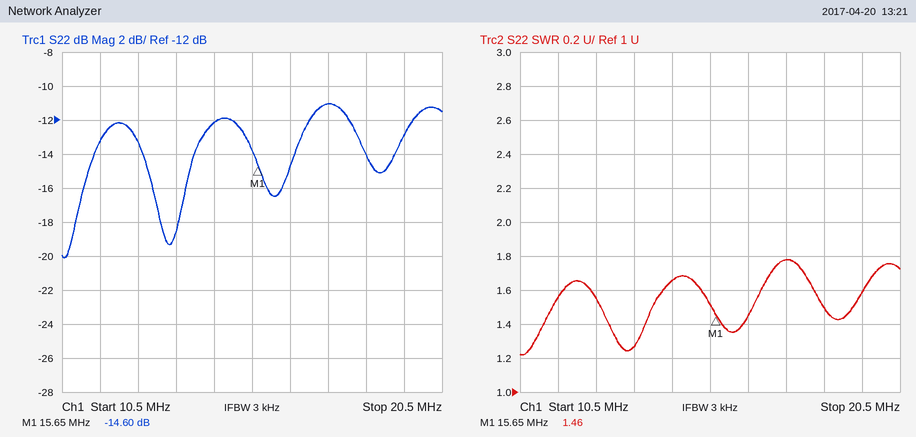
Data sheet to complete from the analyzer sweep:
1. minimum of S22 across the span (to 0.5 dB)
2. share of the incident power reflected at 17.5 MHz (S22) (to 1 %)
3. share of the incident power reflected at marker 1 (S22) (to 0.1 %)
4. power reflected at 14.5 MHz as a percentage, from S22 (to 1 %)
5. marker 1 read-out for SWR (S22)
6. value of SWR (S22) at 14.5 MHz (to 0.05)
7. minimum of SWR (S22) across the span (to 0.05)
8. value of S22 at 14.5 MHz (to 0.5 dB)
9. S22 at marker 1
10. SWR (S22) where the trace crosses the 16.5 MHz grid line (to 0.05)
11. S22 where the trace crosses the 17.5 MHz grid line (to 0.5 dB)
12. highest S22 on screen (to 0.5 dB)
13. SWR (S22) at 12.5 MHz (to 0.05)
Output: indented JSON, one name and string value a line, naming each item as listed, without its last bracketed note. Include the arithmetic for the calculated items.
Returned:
{
  "minimum of S22 across the span": "-20.0 dB",
  "share of the incident power reflected at 17.5 MHz (S22)": "10^(-11/10) ≈ 8 %",
  "share of the incident power reflected at marker 1 (S22)": "10^(-14.6/10) ≈ 3.5 %",
  "power reflected at 14.5 MHz as a percentage, from S22": "10^(-12/10) ≈ 6 %",
  "marker 1 read-out for SWR": "1.46",
  "value of SWR (S22) at 14.5 MHz": "1.65",
  "minimum of SWR (S22) across the span": "1.20",
  "value of S22 at 14.5 MHz": "-12.0 dB",
  "S22 at marker 1": "-14.60 dB",
  "SWR (S22) where the trace crosses the 16.5 MHz grid line": "1.45",
  "S22 where the trace crosses the 17.5 MHz grid line": "-11.0 dB",
  "highest S22 on screen": "-11.0 dB",
  "SWR (S22) at 12.5 MHz": "1.55"
}
